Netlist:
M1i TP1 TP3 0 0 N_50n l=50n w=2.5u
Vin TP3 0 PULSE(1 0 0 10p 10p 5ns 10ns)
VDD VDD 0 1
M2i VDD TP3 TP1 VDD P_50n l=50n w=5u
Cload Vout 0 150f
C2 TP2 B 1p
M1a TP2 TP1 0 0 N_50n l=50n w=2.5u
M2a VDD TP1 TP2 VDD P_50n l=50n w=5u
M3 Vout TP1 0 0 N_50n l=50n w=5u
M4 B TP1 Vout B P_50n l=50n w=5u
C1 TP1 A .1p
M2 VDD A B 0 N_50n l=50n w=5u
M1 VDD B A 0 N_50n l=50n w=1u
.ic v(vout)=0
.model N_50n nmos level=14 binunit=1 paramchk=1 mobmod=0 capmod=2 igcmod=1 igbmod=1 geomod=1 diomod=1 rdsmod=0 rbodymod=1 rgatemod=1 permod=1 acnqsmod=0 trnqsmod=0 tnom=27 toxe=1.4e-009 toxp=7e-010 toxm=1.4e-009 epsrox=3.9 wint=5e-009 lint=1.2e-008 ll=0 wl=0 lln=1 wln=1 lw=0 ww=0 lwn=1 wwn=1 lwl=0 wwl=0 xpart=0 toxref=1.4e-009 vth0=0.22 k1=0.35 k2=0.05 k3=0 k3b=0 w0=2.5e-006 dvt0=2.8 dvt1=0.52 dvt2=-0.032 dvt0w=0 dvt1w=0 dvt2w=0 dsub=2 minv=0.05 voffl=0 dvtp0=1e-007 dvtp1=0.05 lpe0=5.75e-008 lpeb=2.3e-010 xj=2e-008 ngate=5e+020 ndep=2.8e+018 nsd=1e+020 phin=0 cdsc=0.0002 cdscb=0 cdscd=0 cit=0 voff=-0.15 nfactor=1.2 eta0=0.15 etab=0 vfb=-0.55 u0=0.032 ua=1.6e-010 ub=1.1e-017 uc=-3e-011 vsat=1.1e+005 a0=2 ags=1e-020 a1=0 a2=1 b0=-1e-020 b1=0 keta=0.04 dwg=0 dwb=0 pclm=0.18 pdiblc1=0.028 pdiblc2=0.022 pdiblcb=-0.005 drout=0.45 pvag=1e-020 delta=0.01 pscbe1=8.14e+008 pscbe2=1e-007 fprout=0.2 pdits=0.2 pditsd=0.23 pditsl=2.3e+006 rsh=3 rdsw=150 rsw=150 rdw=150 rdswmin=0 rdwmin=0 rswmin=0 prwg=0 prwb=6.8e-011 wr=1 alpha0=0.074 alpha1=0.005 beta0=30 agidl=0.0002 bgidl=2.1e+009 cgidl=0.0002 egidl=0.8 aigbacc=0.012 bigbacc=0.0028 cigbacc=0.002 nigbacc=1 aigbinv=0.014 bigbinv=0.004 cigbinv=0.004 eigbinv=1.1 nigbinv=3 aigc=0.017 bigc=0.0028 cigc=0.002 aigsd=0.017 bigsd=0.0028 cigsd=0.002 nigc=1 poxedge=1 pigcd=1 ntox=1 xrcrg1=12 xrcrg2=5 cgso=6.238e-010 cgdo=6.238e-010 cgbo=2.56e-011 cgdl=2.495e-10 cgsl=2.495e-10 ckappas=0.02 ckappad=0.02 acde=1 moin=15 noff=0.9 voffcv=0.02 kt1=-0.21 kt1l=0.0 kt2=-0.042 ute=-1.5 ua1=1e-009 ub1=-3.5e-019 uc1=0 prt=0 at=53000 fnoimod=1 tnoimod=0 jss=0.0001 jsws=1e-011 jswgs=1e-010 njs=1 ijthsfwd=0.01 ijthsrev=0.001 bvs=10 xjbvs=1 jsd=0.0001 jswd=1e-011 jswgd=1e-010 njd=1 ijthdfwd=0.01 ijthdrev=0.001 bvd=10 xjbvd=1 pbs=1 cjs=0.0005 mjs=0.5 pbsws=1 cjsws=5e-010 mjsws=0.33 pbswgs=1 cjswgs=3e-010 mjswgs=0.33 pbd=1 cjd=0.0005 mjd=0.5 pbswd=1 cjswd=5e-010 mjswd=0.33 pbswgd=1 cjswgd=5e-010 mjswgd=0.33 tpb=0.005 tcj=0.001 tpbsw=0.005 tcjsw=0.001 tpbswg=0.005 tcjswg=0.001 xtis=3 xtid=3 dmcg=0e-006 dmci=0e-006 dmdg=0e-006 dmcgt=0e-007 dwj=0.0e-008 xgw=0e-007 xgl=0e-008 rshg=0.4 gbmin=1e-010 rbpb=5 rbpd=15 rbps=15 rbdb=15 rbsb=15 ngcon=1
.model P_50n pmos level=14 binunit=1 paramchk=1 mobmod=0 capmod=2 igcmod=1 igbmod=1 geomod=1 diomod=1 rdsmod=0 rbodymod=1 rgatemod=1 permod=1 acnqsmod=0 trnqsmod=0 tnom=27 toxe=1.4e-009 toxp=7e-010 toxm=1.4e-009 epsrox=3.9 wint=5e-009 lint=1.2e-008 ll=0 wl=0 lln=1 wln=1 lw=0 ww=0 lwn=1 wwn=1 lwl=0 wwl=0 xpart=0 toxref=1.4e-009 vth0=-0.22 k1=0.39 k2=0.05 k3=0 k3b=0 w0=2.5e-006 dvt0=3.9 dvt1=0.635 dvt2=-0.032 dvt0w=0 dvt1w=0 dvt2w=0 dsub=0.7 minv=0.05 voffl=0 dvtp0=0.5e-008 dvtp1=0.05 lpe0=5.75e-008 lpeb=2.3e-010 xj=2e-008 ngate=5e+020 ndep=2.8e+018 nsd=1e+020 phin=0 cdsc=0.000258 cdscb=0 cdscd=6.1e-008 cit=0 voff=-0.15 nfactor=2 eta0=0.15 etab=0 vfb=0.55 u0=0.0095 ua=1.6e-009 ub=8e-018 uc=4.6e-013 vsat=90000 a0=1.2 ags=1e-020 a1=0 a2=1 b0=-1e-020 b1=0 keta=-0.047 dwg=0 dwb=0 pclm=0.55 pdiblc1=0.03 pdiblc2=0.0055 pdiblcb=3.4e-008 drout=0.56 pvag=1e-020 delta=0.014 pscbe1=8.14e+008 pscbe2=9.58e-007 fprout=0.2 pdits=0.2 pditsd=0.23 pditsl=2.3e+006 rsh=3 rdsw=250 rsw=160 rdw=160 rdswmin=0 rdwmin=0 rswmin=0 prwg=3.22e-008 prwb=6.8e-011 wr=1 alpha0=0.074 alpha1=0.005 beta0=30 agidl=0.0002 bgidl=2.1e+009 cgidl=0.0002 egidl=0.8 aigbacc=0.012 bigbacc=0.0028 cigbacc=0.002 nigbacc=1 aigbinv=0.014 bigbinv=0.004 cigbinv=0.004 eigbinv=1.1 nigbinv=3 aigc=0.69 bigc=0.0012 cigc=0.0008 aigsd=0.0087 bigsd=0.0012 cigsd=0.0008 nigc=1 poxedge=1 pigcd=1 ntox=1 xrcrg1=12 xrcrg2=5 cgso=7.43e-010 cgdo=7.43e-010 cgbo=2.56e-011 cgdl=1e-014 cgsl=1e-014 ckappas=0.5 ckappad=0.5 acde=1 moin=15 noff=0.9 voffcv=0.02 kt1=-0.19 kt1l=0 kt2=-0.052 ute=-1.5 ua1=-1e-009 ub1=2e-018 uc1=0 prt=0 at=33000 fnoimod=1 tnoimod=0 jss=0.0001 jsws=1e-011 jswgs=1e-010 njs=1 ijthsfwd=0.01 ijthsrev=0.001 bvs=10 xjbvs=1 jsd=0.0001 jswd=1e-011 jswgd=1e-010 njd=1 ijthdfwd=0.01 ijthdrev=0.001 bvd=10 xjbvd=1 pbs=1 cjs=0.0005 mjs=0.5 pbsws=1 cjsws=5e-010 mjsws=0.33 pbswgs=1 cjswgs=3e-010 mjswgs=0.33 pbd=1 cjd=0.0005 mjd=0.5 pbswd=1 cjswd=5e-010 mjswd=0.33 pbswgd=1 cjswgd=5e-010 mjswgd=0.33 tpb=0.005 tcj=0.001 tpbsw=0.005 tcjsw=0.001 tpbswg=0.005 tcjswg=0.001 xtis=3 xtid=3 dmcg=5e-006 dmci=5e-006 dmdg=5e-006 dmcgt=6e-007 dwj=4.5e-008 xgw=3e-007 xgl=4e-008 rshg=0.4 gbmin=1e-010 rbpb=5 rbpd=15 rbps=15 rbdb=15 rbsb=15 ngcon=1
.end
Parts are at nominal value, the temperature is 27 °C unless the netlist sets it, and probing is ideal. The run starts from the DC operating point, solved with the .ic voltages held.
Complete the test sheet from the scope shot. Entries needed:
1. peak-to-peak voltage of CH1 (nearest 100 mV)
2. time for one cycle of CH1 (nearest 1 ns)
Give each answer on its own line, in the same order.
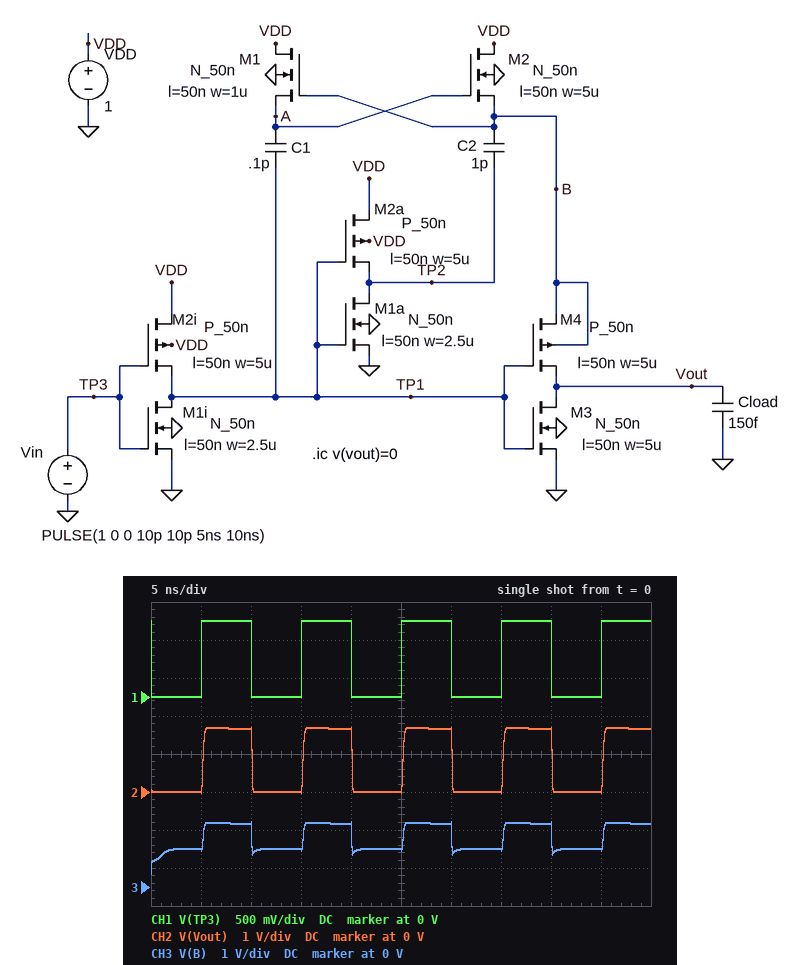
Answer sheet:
1.0 V
10 ns
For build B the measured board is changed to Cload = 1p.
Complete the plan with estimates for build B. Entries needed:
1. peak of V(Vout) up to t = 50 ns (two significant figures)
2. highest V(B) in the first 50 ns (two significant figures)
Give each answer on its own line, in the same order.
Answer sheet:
990 mV
1.0 V
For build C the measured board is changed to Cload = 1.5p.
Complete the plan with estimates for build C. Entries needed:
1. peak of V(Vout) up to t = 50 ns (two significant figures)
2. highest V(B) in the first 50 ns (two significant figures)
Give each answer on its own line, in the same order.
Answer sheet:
790 mV
1.0 V
